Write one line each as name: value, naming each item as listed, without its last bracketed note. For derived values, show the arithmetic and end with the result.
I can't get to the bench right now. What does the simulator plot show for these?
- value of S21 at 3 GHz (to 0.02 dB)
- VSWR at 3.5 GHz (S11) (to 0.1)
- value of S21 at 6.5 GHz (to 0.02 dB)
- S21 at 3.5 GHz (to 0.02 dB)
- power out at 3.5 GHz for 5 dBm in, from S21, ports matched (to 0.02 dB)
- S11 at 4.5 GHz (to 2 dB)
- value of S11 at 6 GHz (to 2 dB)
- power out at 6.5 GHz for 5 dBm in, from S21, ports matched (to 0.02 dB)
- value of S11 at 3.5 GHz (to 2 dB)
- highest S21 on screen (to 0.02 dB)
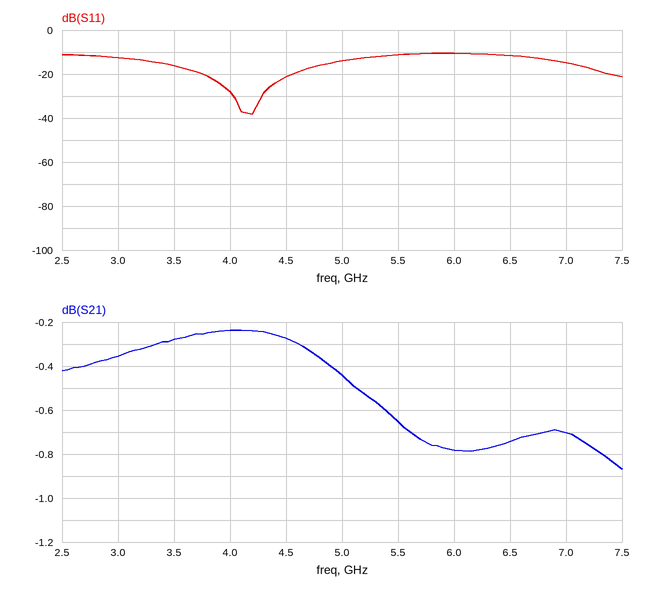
value of S21 at 3 GHz: -0.36 dB
VSWR at 3.5 GHz (S11): |Γ| = 10^(-16/20) = 0.1585; VSWR = (1 + 0.1585)/(1 − 0.1585) ≈ 1.4
value of S21 at 6.5 GHz: -0.74 dB
S21 at 3.5 GHz: -0.28 dB
power out at 3.5 GHz for 5 dBm in, from S21, ports matched: 5 dBm + (-0.28 dB) = 4.72 dBm
S11 at 4.5 GHz: -22 dB
value of S11 at 6 GHz: -10 dB
power out at 6.5 GHz for 5 dBm in, from S21, ports matched: 5 dBm + (-0.74 dB) = 4.26 dBm
value of S11 at 3.5 GHz: -16 dB
highest S21 on screen: -0.24 dB
